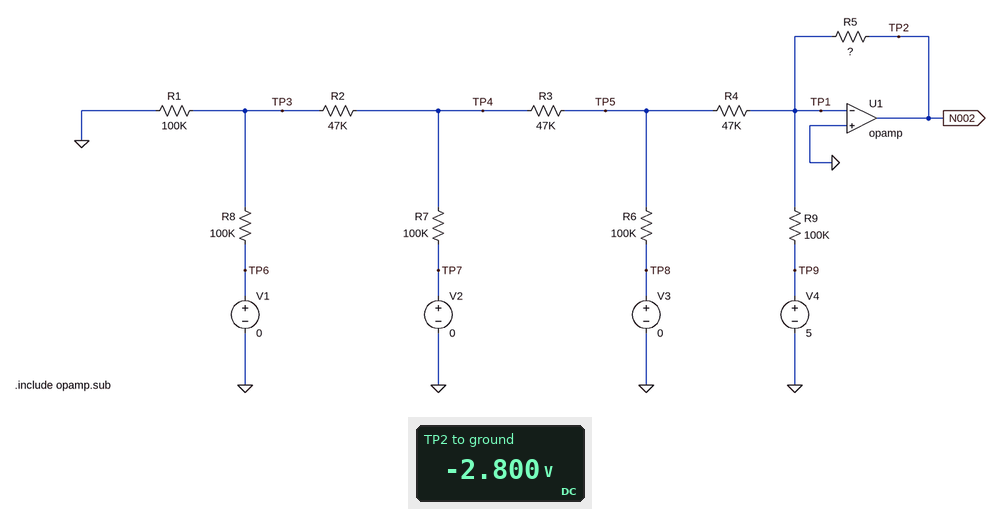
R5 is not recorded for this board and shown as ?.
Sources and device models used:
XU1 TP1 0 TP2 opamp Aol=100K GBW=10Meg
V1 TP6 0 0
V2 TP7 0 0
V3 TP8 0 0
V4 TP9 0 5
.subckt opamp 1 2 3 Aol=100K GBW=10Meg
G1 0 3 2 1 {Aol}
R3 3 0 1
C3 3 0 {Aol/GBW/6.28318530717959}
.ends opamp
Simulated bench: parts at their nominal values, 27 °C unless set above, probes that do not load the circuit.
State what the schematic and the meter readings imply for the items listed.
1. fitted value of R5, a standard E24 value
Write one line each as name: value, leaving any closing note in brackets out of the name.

fitted value of R5, a standard E24 value: 56 kΩ
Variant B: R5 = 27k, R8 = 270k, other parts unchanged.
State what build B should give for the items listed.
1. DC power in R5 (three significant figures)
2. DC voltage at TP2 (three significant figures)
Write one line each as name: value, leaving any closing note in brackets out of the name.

DC power in R5: 67.5 µW
DC voltage at TP2: -1.35 V
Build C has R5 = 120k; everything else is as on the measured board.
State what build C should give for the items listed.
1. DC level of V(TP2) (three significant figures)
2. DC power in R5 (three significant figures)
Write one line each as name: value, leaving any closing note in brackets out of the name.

DC level of V(TP2): -6.00 V
DC power in R5: 300 µW
